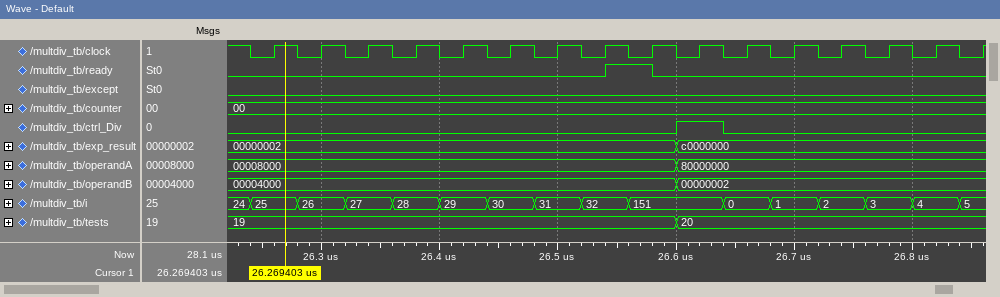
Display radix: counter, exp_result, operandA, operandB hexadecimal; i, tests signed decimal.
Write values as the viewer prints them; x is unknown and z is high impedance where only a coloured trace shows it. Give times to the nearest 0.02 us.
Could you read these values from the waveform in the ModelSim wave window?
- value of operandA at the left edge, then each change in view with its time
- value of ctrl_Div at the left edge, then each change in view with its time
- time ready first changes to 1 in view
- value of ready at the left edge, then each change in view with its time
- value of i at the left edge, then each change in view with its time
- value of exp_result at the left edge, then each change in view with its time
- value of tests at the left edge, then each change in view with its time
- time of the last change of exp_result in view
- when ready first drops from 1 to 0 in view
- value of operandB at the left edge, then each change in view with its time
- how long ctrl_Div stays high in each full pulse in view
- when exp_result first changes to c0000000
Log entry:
00008000, 80000000 at 26.6 us
0, 1 at 26.6 us, 0 at 26.64 us
26.54 us
0, 1 at 26.54 us, 0 at 26.58 us
24, 25 at 26.24 us, 26 at 26.28 us, 27 at 26.32 us, 28 at 26.36 us, 29 at 26.4 us, 30 at 26.44 us, 31 at 26.48 us, 32 at 26.52 us, 151 at 26.56 us, 0 at 26.64 us, 1 at 26.68 us, 2 at 26.72 us, 3 at 26.76 us, 4 at 26.8 us, 5 at 26.84 us
00000002, c0000000 at 26.6 us
19, 20 at 26.6 us
26.6 us
26.58 us
00004000, 00000002 at 26.6 us
0.04 us
26.6 us
